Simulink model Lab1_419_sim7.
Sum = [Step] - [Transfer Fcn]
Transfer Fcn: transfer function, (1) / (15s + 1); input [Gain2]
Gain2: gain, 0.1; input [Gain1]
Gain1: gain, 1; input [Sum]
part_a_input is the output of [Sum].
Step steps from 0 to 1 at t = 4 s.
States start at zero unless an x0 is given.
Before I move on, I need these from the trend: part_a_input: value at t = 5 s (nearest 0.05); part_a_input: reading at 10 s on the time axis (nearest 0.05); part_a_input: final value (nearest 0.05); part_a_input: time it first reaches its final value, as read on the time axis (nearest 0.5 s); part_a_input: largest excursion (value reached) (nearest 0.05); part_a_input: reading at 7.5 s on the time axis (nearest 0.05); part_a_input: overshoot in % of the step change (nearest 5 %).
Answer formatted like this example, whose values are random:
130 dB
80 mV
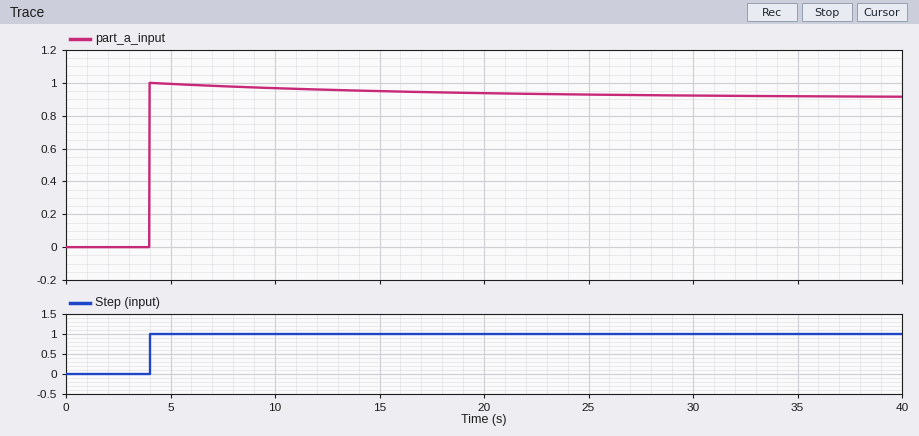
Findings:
1.00
0.95
0.90
4.0 s
1.00
1.00
10 %
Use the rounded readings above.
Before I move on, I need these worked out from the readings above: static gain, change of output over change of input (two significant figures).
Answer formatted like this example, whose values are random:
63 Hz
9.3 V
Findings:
0.90
